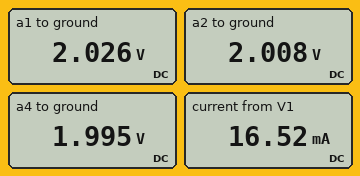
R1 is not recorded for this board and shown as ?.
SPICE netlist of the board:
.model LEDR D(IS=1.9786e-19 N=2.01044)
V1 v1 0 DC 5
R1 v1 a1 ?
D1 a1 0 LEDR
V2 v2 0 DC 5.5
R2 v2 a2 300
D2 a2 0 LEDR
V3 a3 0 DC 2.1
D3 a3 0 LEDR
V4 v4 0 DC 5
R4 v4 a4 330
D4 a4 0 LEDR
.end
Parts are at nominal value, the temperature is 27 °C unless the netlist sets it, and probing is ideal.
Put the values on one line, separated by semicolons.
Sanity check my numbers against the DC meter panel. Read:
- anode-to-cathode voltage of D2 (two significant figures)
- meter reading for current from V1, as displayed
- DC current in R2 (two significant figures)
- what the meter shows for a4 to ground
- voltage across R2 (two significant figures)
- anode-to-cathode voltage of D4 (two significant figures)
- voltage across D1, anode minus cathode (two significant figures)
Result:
2.0 V; 16.52 mA; 12 mA; 1.995 V; 3.5 V; 2.0 V; 2.0 V
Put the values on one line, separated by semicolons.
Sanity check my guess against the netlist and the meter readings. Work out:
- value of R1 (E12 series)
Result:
180 Ω
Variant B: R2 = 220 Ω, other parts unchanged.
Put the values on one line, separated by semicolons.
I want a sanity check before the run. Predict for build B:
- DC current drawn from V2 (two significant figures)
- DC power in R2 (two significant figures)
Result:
16 mA; 55 mW
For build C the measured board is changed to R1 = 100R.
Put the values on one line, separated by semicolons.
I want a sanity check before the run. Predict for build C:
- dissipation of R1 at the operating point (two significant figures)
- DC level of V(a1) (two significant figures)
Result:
87 mW; 2.1 V
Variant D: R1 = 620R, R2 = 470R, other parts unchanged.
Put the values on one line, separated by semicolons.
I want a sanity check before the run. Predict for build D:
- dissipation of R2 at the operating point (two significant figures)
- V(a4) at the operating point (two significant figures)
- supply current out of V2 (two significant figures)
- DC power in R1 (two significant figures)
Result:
26 mW; 2.0 V; 7.5 mA; 15 mW
